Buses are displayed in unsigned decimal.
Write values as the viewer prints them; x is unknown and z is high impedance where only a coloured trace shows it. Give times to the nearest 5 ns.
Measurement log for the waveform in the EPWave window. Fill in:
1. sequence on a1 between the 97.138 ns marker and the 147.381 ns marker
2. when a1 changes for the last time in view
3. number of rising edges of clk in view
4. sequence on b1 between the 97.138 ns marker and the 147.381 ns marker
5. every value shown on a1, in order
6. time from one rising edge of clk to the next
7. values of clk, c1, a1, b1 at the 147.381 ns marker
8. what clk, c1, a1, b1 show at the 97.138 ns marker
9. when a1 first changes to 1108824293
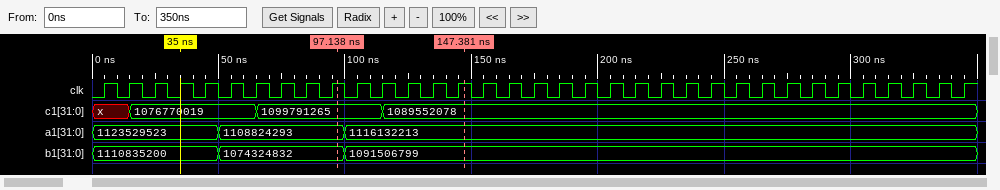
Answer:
1108824293, 1116132213
100 ns
35
1074324832, 1091506799
1123529523, 1108824293, 1116132213
10 ns
clk=1, c1=1089552078, a1=1116132213, b1=1091506799
clk=1, c1=1099791265, a1=1108824293, b1=1074324832
50 ns
